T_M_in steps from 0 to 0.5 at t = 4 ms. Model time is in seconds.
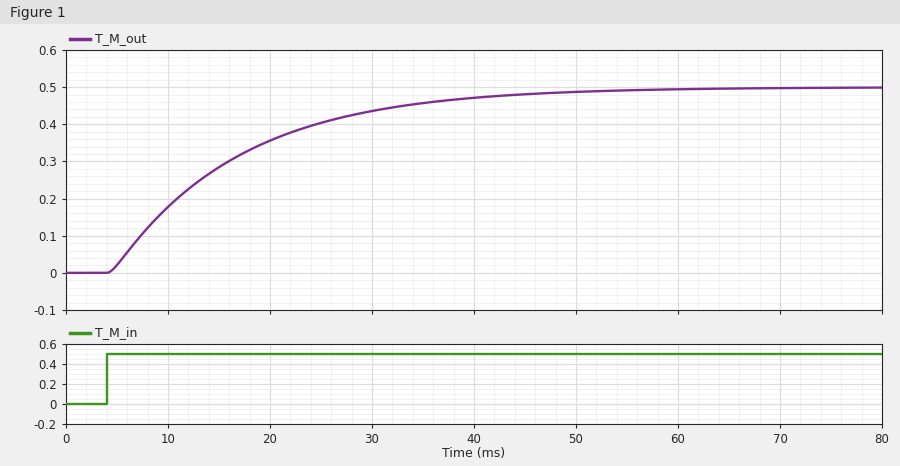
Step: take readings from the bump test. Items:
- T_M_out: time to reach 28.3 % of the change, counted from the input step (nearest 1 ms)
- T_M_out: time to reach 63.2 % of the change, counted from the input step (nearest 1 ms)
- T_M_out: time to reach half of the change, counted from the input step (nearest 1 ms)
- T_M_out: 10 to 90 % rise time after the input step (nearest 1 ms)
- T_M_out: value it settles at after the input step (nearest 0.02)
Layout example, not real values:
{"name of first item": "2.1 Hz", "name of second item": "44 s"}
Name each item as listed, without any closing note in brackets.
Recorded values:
{"T_M_out: time to reach 28.3 % of the change, counted from the input step": "5 ms", "T_M_out: time to reach 63.2 % of the change, counted from the input step": "13 ms", "T_M_out: time to reach half of the change, counted from the input step": "9 ms", "T_M_out: 10 to 90 % rise time after the input step": "27 ms", "T_M_out: value it settles at after the input step": "0.50"}
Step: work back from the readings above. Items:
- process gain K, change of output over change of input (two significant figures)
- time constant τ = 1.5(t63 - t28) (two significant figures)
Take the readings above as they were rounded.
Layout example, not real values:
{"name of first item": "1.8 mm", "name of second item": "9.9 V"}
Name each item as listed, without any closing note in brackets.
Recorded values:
{"process gain K, change of output over change of input": "1.0", "time constant τ = 1.5(t63 - t28)": "12 ms"}
